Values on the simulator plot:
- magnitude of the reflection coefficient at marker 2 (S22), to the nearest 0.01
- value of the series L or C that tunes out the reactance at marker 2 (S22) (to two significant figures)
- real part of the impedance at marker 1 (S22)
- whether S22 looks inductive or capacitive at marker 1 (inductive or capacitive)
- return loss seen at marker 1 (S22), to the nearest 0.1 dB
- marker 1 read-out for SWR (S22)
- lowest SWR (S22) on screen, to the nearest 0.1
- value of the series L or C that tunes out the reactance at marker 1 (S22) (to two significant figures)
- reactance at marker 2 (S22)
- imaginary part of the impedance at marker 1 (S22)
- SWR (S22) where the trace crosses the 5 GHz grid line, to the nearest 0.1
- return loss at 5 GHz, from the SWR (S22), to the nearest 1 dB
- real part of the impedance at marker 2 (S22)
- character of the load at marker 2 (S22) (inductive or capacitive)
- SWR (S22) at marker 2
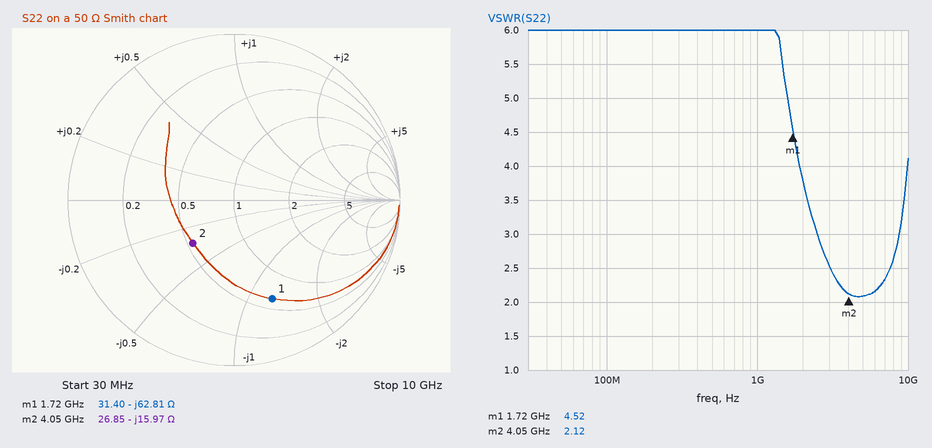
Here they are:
0.36
630 pH
31.40 Ω
capacitive
3.9 dB
4.52
2.1
5.8 nH
-15.97 Ω
-62.81 Ω
2.1
9 dB
26.85 Ω
capacitive
2.12
